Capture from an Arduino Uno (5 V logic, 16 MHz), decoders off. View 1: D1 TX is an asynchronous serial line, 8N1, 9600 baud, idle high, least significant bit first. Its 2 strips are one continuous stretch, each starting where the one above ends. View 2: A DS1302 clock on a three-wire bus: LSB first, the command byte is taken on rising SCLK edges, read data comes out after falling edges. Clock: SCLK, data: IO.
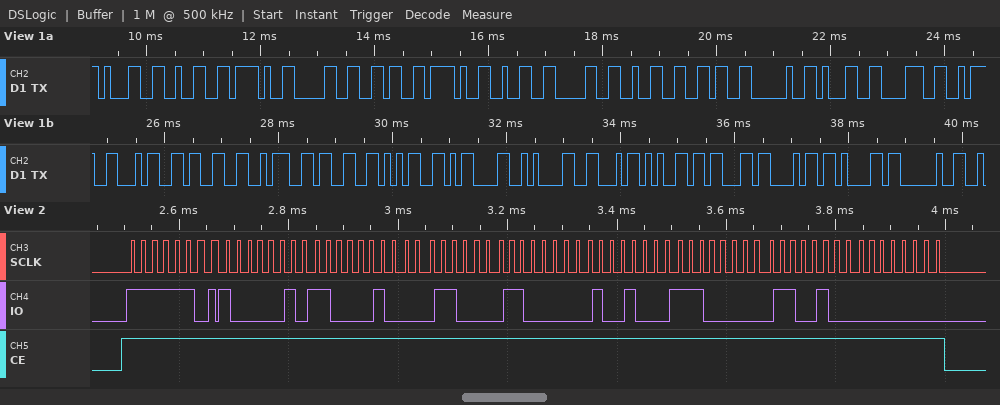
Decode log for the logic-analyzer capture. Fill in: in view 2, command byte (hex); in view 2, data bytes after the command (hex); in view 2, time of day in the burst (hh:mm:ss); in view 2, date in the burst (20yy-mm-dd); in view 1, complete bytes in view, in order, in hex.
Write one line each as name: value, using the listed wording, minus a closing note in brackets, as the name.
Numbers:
in view 2, command byte: 0xBF
in view 2, data bytes after the command: 41 43 18 06 12 07 26 00
in view 2, time of day in the burst: 18:43:41
in view 2, date in the burst: 2026-12-06
in view 1, complete bytes in view, in order, in hex: 31 32 2F 30 36 2F 32 30 32 36 20 31 38 3A 34 33 3A 33 35 0D 0A 46 65 63 68 61 20
